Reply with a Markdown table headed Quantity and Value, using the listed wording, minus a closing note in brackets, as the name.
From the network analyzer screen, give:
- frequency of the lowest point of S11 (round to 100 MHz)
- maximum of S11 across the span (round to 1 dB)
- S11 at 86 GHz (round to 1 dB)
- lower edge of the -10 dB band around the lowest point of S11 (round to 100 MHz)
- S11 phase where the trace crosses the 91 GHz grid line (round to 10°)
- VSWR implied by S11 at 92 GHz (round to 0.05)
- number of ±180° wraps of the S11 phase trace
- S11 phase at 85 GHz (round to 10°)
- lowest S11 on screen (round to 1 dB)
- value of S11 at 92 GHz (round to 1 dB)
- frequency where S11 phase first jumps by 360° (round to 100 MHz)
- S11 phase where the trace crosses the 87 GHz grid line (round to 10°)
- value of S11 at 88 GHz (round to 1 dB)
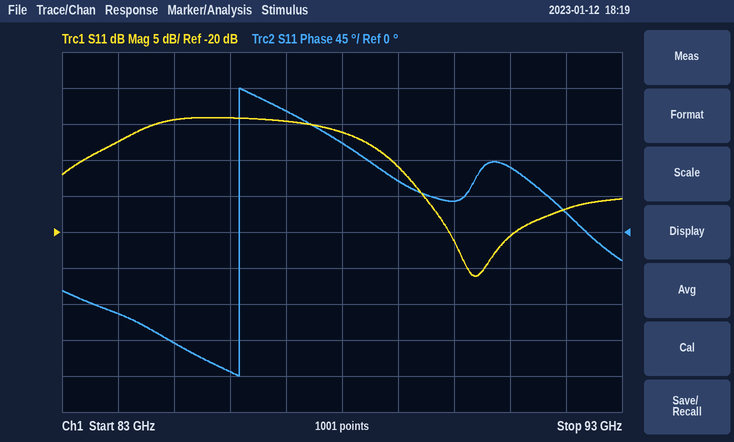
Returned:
| Quantity | Value |
|---|---|
| frequency of the lowest point of S11 | 90.4 GHz |
| maximum of S11 across the span | -4 dB |
| S11 at 86 GHz | -4 dB |
| lower edge of the -10 dB band around the lowest point of S11 | 88.9 GHz |
| S11 phase where the trace crosses the 91 GHz grid line | 80° |
| VSWR implied by S11 at 92 GHz | 1.35 |
| number of ±180° wraps of the S11 phase trace | 1 |
| S11 phase at 85 GHz | -140° |
| lowest S11 on screen | -26 dB |
| value of S11 at 92 GHz | -17 dB |
| frequency where S11 phase first jumps by 360° | 86.2 GHz |
| S11 phase where the trace crosses the 87 GHz grid line | 150° |
| value of S11 at 88 GHz | -6 dB |
